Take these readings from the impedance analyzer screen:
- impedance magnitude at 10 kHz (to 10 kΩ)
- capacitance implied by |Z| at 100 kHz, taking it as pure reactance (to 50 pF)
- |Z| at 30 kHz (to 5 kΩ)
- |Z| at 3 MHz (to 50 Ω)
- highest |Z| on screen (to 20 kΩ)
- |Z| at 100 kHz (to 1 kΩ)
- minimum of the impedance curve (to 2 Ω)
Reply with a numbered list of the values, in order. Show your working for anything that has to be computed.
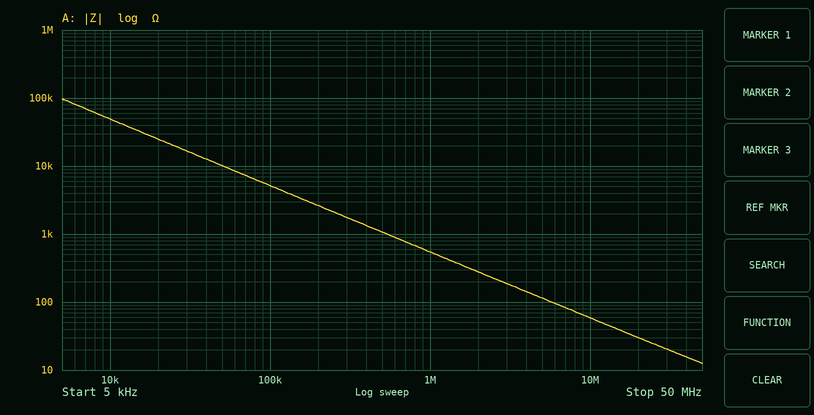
1. 50 kΩ
2. C = 1/(2π × 100 kHz × 5 kΩ) ≈ 318 pF, so 300 pF to the nearest 50 pF
3. 15 kΩ
4. 200 Ω
5. 100 kΩ
6. 5 kΩ
7. 12 Ω
